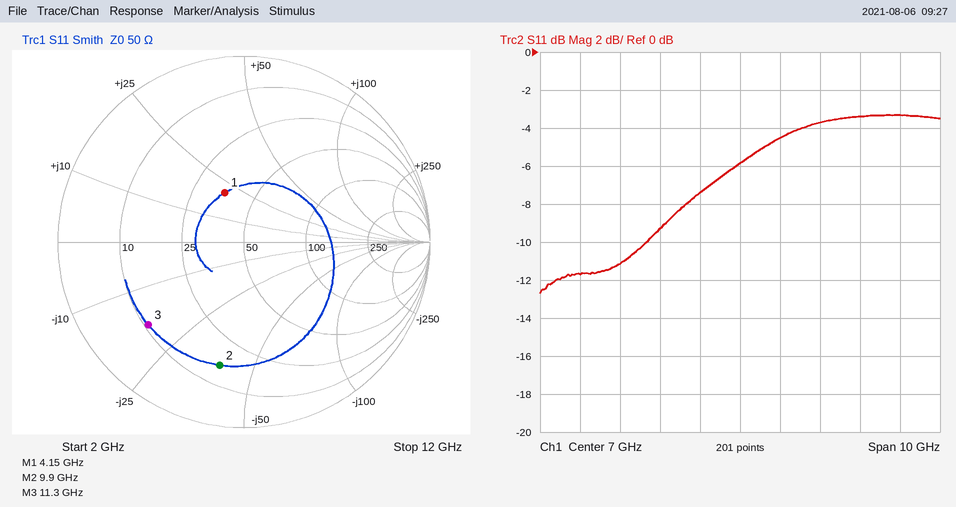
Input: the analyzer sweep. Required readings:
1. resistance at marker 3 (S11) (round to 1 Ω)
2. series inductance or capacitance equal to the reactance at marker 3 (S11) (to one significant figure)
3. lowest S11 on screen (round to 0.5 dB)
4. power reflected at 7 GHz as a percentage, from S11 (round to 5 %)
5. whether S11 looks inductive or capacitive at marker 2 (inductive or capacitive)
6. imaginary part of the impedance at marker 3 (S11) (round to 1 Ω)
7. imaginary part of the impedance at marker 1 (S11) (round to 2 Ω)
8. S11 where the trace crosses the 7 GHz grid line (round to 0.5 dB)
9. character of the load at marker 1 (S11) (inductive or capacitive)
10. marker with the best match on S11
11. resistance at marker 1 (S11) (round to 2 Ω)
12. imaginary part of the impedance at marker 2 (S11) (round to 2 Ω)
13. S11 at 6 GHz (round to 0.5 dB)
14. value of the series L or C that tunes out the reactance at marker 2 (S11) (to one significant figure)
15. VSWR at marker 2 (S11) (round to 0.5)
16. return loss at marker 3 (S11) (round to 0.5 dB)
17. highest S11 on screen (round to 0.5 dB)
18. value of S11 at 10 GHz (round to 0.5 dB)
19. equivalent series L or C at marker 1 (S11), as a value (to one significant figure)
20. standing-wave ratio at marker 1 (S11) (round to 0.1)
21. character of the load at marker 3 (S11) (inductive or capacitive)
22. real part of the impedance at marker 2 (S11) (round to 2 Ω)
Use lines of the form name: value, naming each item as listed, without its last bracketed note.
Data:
resistance at marker 3 (S11): 11 Ω
series inductance or capacitance equal to the reactance at marker 3 (S11): 800 fF
lowest S11 on screen: -12.5 dB
power reflected at 7 GHz as a percentage, from S11: 25 %
whether S11 looks inductive or capacitive at marker 2: capacitive
imaginary part of the impedance at marker 3 (S11): -18 Ω
imaginary part of the impedance at marker 1 (S11): +20 Ω
S11 where the trace crosses the 7 GHz grid line: -6.0 dB
character of the load at marker 1 (S11): inductive
marker with the best match on S11: marker 1
resistance at marker 1 (S11): 36 Ω
imaginary part of the impedance at marker 2 (S11): -38 Ω
S11 at 6 GHz: -7.5 dB
value of the series L or C that tunes out the reactance at marker 2 (S11): 600 pH
VSWR at marker 2 (S11): 5.0
return loss at marker 3 (S11): 3.5 dB
highest S11 on screen: -3.5 dB
value of S11 at 10 GHz: -3.5 dB
equivalent series L or C at marker 1 (S11), as a value: 800 pH
standing-wave ratio at marker 1 (S11): 1.8
character of the load at marker 3 (S11): capacitive
real part of the impedance at marker 2 (S11): 16 Ω
